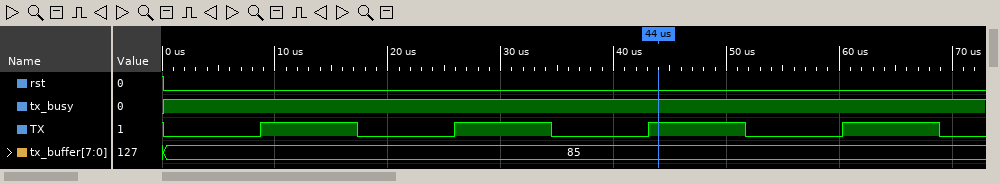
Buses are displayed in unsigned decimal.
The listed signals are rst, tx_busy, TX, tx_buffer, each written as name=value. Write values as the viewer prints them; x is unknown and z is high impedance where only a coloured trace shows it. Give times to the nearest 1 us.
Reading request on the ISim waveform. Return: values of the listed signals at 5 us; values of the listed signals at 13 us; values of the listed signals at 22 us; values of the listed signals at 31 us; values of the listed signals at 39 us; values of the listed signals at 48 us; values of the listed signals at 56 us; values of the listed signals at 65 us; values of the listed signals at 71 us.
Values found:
rst=0, tx_busy=1, TX=0, tx_buffer=85
rst=0, tx_busy=1, TX=1, tx_buffer=85
rst=0, tx_busy=1, TX=0, tx_buffer=85
rst=0, tx_busy=1, TX=1, tx_buffer=85
rst=0, tx_busy=1, TX=0, tx_buffer=85
rst=0, tx_busy=1, TX=1, tx_buffer=85
rst=0, tx_busy=1, TX=0, tx_buffer=85
rst=0, tx_busy=1, TX=1, tx_buffer=85
rst=0, tx_busy=1, TX=0, tx_buffer=85
